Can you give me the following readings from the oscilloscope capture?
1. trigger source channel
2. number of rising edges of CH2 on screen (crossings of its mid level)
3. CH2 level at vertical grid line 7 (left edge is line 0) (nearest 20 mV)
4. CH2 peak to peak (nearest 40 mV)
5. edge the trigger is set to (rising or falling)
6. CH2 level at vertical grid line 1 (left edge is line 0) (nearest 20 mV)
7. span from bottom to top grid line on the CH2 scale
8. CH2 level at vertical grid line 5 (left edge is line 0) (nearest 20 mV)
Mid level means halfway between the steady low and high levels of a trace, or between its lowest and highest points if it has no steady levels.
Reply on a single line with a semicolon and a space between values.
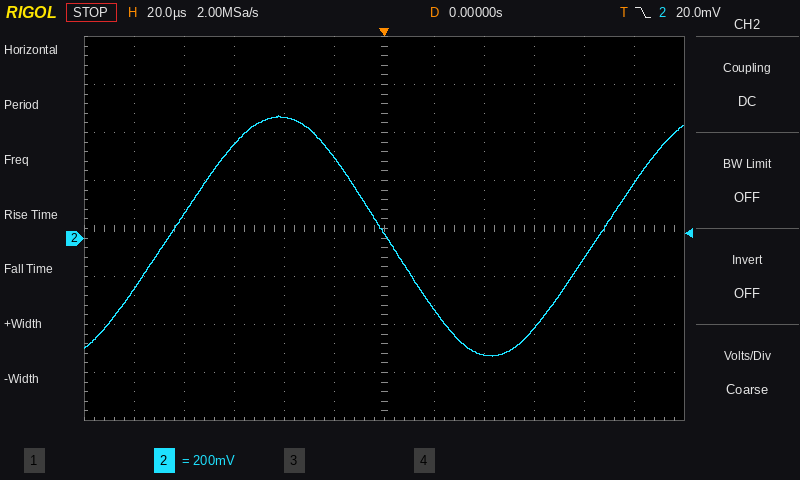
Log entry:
CH2; 2; -300 mV; 1.00 V; falling; -220 mV; 1.6 V; 340 mV
